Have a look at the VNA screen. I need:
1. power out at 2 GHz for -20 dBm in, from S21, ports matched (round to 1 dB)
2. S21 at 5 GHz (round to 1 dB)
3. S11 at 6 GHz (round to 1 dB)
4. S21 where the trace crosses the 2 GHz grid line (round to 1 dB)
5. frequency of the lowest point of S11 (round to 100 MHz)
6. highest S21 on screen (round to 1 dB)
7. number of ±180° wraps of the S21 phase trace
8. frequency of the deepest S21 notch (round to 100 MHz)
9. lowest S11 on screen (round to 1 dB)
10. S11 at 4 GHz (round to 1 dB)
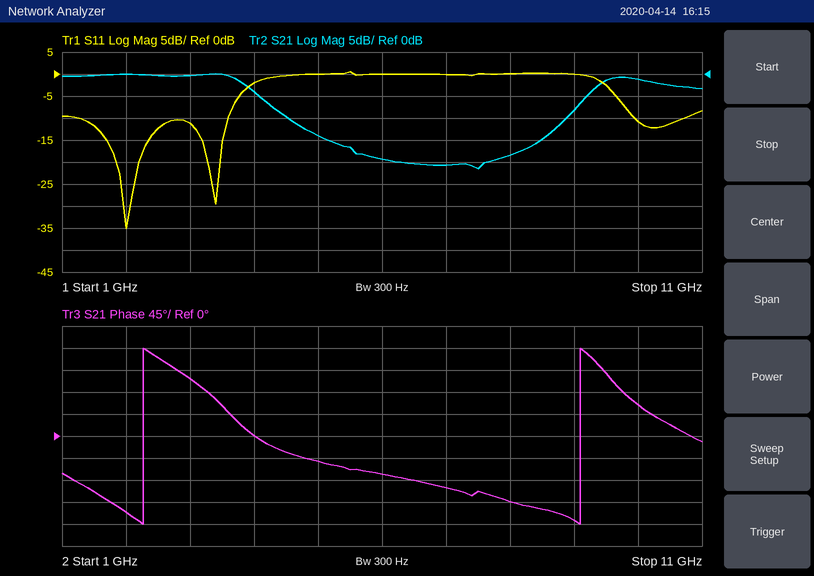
-20 dBm
-14 dB
0 dB
0 dB
2.0 GHz
0 dB
2
7.5 GHz
-35 dB
-2 dB
